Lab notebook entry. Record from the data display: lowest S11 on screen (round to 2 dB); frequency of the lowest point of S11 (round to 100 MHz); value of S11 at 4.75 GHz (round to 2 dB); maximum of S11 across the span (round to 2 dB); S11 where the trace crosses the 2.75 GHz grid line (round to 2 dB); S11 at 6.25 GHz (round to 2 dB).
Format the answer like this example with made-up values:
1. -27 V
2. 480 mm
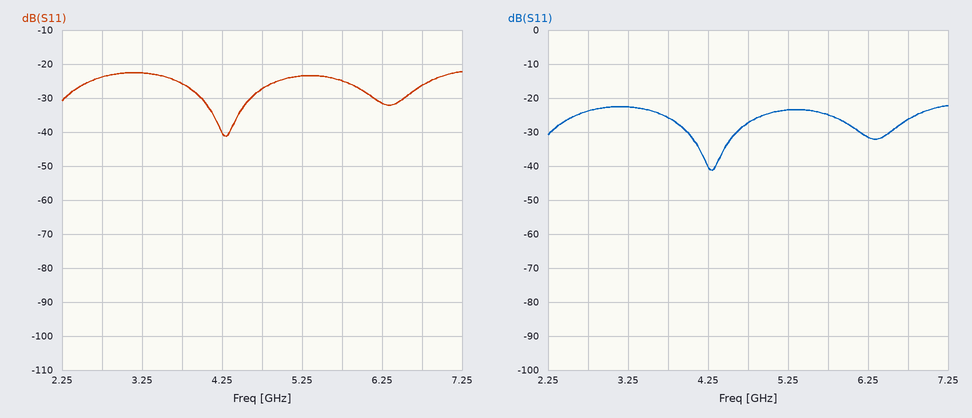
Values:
1. -42 dB
2. 4.3 GHz
3. -28 dB
4. -22 dB
5. -24 dB
6. -32 dB
